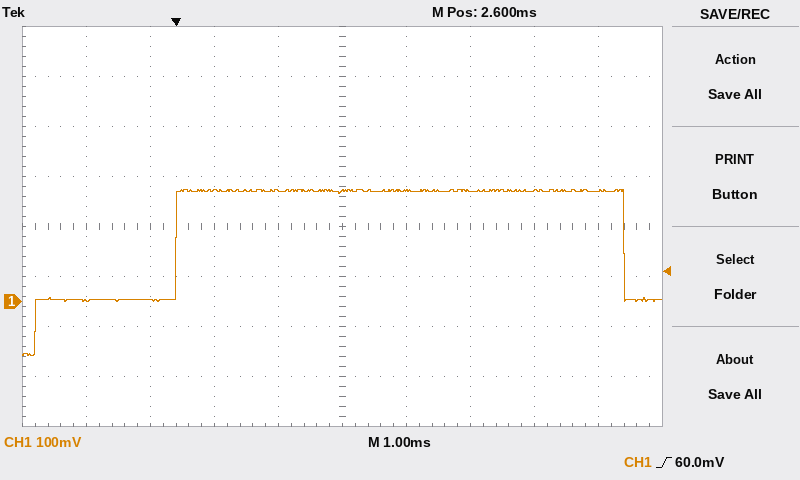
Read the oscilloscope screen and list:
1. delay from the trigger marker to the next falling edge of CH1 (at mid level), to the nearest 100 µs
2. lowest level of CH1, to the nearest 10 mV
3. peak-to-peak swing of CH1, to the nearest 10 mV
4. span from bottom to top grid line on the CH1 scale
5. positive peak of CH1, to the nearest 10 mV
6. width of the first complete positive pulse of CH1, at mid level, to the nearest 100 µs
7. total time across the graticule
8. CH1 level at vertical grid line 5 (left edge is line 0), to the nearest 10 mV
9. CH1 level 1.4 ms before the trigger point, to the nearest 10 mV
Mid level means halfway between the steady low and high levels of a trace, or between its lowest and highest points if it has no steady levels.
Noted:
7.0 ms
-110 mV
330 mV
800 mV
220 mV
7.0 ms
10 ms
220 mV
0 mV
